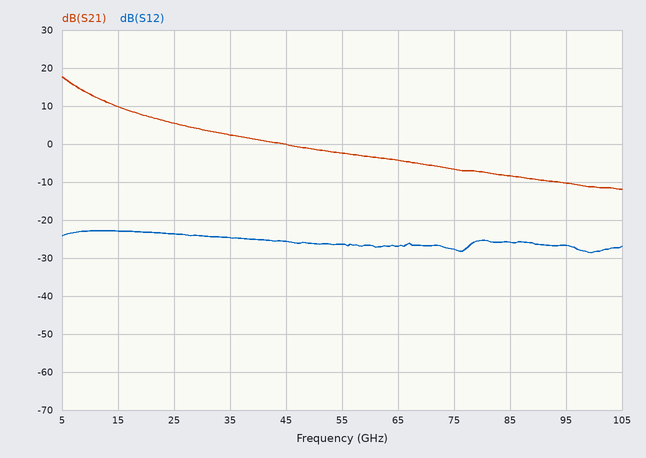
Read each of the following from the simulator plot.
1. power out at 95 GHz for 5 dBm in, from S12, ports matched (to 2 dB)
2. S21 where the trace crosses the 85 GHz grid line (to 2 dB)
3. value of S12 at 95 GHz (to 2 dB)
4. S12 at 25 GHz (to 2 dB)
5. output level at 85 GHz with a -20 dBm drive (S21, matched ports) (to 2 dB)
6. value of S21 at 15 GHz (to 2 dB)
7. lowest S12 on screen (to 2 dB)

-22 dBm
-8 dB
-26 dB
-24 dB
-28 dBm
10 dB
-28 dB
